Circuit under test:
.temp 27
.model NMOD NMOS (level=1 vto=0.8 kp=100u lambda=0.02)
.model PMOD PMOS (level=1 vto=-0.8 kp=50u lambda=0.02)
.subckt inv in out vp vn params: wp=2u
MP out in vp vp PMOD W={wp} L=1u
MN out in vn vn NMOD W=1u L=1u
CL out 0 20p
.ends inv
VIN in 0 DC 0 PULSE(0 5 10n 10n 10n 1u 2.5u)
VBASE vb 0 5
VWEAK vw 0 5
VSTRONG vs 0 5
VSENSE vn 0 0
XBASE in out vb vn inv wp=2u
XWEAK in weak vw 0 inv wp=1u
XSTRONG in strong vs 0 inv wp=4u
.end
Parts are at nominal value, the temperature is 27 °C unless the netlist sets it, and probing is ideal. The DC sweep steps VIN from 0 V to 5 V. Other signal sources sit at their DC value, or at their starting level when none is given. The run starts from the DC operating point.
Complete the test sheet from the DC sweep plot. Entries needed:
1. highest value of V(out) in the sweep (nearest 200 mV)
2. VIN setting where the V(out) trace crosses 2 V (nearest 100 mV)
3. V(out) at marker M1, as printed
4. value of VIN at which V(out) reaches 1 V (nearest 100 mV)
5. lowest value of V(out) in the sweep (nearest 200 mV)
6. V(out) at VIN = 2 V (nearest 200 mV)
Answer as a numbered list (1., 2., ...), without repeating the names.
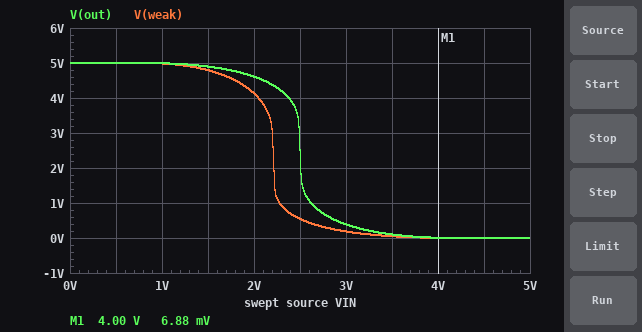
1. 5.0 V
2. 2.5 V
3. 6.88 mV
4. 2.6 V
5. 0 V
6. 4.6 V
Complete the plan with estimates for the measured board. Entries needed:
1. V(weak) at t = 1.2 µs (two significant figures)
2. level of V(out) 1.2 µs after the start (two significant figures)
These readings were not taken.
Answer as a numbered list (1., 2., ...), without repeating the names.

1. 3.5 V
2. 4.7 V
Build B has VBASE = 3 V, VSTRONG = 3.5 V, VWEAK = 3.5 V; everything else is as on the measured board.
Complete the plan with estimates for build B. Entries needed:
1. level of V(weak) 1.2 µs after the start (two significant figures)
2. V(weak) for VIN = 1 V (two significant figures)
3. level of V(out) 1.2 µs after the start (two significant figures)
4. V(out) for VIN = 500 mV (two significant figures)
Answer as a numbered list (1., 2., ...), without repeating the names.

1. 1.6 V
2. 3.5 V
3. 2.0 V
4. 3.0 V
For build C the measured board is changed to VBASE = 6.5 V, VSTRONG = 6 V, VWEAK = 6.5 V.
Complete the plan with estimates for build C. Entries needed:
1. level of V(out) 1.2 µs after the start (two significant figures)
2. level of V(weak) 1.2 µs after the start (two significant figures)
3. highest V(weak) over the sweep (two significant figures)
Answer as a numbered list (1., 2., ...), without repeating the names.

1. 6.4 V
2. 5.5 V
3. 6.5 V
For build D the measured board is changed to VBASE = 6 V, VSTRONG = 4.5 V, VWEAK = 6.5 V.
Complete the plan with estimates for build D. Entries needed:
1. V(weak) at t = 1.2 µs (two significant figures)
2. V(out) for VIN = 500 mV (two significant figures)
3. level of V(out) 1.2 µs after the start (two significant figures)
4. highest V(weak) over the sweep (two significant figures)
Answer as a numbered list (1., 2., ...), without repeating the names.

1. 5.5 V
2. 6.0 V
3. 5.9 V
4. 6.5 V
